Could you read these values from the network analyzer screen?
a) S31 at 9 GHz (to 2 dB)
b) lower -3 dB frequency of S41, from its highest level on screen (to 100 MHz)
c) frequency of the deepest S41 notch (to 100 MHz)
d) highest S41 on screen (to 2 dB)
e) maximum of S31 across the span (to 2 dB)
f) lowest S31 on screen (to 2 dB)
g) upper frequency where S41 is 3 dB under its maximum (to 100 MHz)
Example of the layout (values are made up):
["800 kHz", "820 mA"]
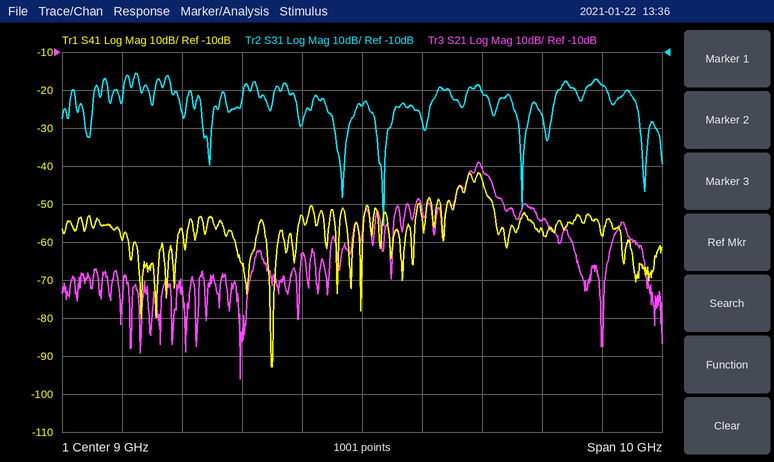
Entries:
["-24 dB", "10.7 GHz", "7.5 GHz", "-42 dB", "-16 dB", "-56 dB", "11.0 GHz"]
